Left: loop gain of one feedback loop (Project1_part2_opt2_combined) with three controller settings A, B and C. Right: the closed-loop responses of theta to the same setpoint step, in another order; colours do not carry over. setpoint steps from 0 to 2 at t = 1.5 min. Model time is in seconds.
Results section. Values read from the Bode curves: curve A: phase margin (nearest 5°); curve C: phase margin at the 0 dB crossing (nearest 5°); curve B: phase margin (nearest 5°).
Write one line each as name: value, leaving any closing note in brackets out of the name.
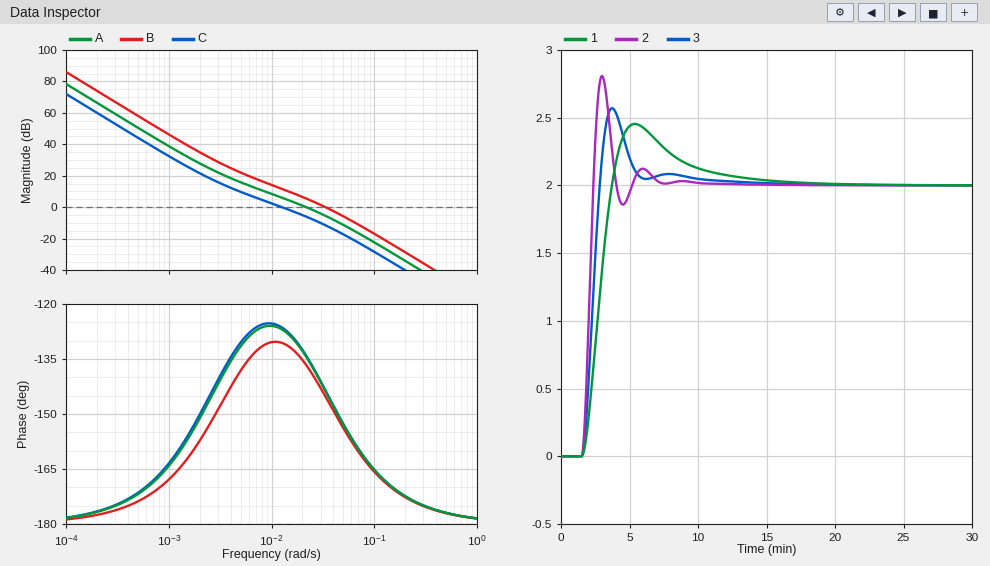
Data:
curve A: phase margin: 45°
curve C: phase margin at the 0 dB crossing: 55°
curve B: phase margin: 35°
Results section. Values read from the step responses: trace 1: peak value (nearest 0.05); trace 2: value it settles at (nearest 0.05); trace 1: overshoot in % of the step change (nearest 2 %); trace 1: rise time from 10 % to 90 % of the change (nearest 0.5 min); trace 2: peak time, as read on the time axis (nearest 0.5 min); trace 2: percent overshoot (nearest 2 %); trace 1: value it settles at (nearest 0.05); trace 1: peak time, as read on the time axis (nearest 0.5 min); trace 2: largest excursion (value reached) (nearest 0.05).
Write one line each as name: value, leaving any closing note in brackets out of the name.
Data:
trace 1: peak value: 2.45
trace 2: value it settles at: 2.00
trace 1: overshoot in % of the step change: 22 %
trace 1: rise time from 10 % to 90 % of the change: 1.5 min
trace 2: peak time, as read on the time axis: 3.0 min
trace 2: percent overshoot: 40 %
trace 1: value it settles at: 2.00
trace 1: peak time, as read on the time axis: 5.5 min
trace 2: largest excursion (value reached): 2.80
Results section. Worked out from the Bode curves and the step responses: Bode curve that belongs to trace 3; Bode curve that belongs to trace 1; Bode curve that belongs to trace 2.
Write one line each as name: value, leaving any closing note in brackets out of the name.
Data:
Bode curve that belongs to trace 3: A
Bode curve that belongs to trace 1: C
Bode curve that belongs to trace 2: B
